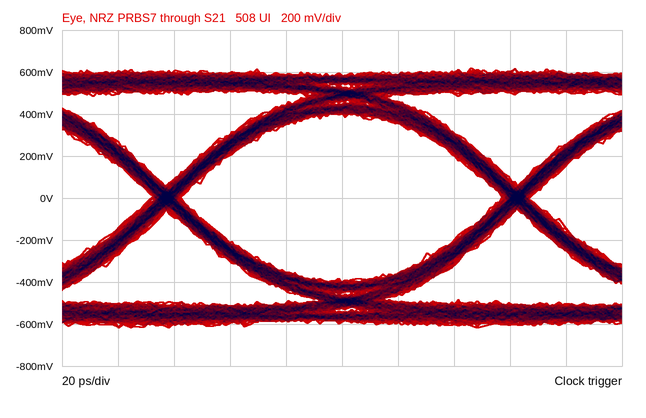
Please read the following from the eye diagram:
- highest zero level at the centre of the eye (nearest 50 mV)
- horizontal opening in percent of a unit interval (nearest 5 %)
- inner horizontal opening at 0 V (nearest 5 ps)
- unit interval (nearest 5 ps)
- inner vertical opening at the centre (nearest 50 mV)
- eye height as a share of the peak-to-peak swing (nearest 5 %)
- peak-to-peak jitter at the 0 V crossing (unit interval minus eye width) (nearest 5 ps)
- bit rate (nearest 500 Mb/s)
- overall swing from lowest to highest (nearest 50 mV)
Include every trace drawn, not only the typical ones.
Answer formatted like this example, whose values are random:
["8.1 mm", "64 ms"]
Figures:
["-400 mV", "90 %", "115 ps", "125 ps", "800 mV", "65 %", "10 ps", "8.0 Gb/s", "1.25 V"]
